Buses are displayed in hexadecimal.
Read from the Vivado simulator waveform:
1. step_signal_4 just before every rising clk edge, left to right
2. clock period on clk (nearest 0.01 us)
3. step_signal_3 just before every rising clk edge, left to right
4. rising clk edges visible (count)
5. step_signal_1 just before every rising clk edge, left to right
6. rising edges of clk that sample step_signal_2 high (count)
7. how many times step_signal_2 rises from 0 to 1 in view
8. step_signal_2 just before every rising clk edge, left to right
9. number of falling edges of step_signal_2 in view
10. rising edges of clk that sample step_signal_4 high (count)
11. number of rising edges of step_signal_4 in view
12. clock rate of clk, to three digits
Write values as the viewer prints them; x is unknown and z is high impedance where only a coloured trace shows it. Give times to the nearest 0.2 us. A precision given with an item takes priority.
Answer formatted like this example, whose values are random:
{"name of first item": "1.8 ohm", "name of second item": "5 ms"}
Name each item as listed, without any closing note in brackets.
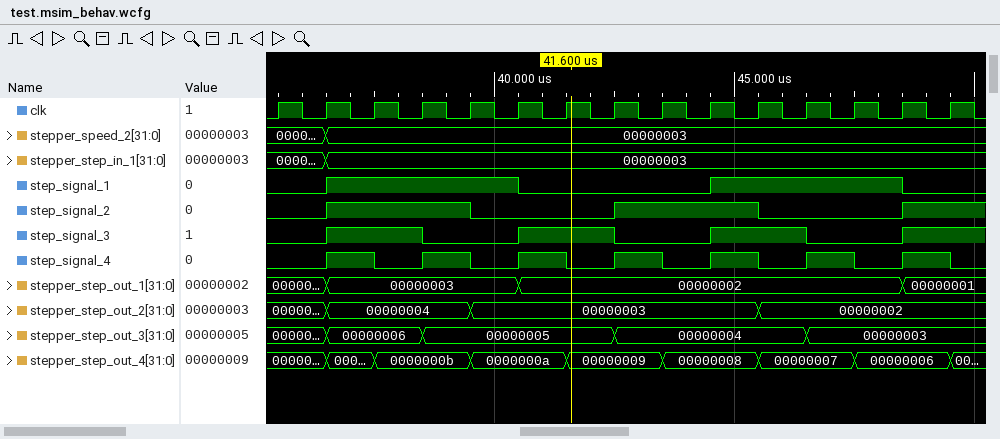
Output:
{"step_signal_4 just before every rising clk edge, left to right": "0 0 1 0 1 0 1 0 1 0 1 0 1 0 1", "clock period on clk": "1 us", "step_signal_3 just before every rising clk edge, left to right": "0 0 1 1 0 0 1 1 0 0 1 1 0 0 1", "rising clk edges visible": "15", "step_signal_1 just before every rising clk edge, left to right": "0 0 1 1 1 1 0 0 0 0 1 1 1 1 0", "rising edges of clk that sample step_signal_2 high": "7", "how many times step_signal_2 rises from 0 to 1 in view": "3", "step_signal_2 just before every rising clk edge, left to right": "0 0 1 1 1 0 0 0 1 1 1 0 0 0 1", "number of falling edges of step_signal_2 in view": "2", "rising edges of clk that sample step_signal_4 high": "7", "number of rising edges of step_signal_4 in view": "7", "clock rate of clk, to three digits": "1.00 MHz"}
